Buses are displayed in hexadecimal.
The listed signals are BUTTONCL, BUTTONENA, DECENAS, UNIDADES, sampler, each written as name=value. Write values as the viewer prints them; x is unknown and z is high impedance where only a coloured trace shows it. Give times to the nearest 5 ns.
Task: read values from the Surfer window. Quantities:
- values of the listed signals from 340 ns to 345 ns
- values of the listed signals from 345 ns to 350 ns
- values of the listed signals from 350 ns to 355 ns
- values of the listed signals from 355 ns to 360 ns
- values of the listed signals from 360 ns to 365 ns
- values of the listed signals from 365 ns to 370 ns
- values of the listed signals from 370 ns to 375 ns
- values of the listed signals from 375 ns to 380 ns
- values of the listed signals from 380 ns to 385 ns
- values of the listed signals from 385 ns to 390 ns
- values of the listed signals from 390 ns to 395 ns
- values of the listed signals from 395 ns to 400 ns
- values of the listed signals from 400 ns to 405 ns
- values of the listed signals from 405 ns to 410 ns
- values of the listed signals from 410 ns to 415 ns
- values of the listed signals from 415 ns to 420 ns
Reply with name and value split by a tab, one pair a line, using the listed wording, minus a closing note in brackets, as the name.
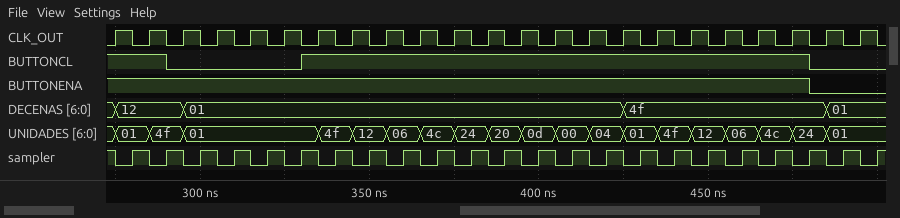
values of the listed signals from 340 ns to 345 ns	BUTTONCL=1, BUTTONENA=1, DECENAS=01, UNIDADES=4f, sampler=1
values of the listed signals from 345 ns to 350 ns	BUTTONCL=1, BUTTONENA=1, DECENAS=01, UNIDADES=12, sampler=0
values of the listed signals from 350 ns to 355 ns	BUTTONCL=1, BUTTONENA=1, DECENAS=01, UNIDADES=12, sampler=1
values of the listed signals from 355 ns to 360 ns	BUTTONCL=1, BUTTONENA=1, DECENAS=01, UNIDADES=06, sampler=0
values of the listed signals from 360 ns to 365 ns	BUTTONCL=1, BUTTONENA=1, DECENAS=01, UNIDADES=06, sampler=1
values of the listed signals from 365 ns to 370 ns	BUTTONCL=1, BUTTONENA=1, DECENAS=01, UNIDADES=4c, sampler=0
values of the listed signals from 370 ns to 375 ns	BUTTONCL=1, BUTTONENA=1, DECENAS=01, UNIDADES=4c, sampler=1
values of the listed signals from 375 ns to 380 ns	BUTTONCL=1, BUTTONENA=1, DECENAS=01, UNIDADES=24, sampler=0
values of the listed signals from 380 ns to 385 ns	BUTTONCL=1, BUTTONENA=1, DECENAS=01, UNIDADES=24, sampler=1
values of the listed signals from 385 ns to 390 ns	BUTTONCL=1, BUTTONENA=1, DECENAS=01, UNIDADES=20, sampler=0
values of the listed signals from 390 ns to 395 ns	BUTTONCL=1, BUTTONENA=1, DECENAS=01, UNIDADES=20, sampler=1
values of the listed signals from 395 ns to 400 ns	BUTTONCL=1, BUTTONENA=1, DECENAS=01, UNIDADES=0d, sampler=0
values of the listed signals from 400 ns to 405 ns	BUTTONCL=1, BUTTONENA=1, DECENAS=01, UNIDADES=0d, sampler=1
values of the listed signals from 405 ns to 410 ns	BUTTONCL=1, BUTTONENA=1, DECENAS=01, UNIDADES=00, sampler=0
values of the listed signals from 410 ns to 415 ns	BUTTONCL=1, BUTTONENA=1, DECENAS=01, UNIDADES=00, sampler=1
values of the listed signals from 415 ns to 420 ns	BUTTONCL=1, BUTTONENA=1, DECENAS=01, UNIDADES=04, sampler=0
